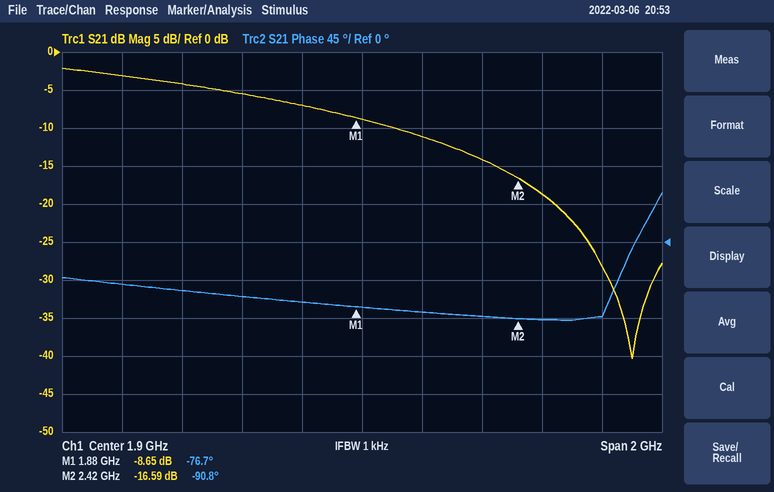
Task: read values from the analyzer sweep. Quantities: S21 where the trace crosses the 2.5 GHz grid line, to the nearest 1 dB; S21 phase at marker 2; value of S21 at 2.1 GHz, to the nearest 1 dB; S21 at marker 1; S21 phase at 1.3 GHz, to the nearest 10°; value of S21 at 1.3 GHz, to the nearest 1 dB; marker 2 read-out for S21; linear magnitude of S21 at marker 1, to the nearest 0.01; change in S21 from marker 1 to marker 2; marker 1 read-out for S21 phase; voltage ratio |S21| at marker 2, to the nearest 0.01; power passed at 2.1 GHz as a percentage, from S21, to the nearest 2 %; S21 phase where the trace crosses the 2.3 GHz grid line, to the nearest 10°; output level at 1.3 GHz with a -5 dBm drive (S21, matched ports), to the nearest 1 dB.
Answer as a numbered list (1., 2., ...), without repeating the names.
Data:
1. -19 dB
2. -90.8°
3. -11 dB
4. -8.65 dB
5. -60°
6. -4 dB
7. -16.59 dB
8. 0.37
9. -7.94 dB
10. -76.7°
11. 0.15
12. 8 %
13. -90°
14. -9 dBm
